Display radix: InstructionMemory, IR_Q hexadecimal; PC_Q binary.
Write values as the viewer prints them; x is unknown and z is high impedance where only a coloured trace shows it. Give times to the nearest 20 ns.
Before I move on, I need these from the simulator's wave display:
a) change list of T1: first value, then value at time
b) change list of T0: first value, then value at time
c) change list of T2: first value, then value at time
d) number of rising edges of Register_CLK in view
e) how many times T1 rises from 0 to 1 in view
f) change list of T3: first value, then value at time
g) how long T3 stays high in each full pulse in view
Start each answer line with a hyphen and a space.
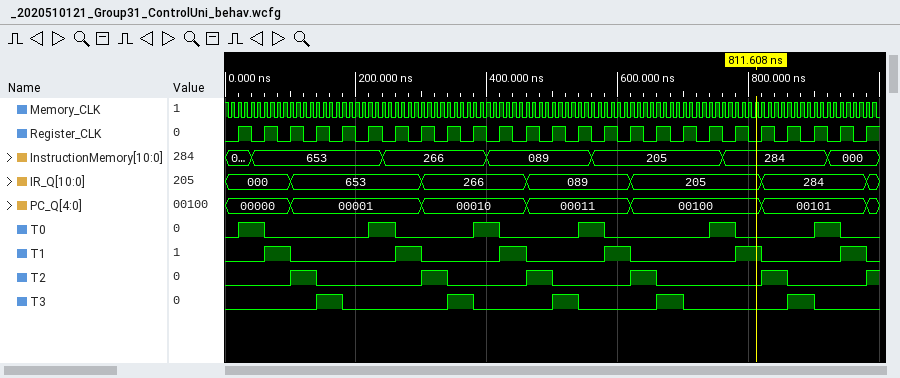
- 0, 1 at 60 ns, 0 at 100 ns, 1 at 260 ns, 0 at 300 ns, 1 at 420 ns, 0 at 460 ns, 1 at 580 ns, 0 at 620 ns, 1 at 780 ns, 0 at 820 ns, 1 at 940 ns, 0 at 980 ns
- 0, 1 at 20 ns, 0 at 60 ns, 1 at 220 ns, 0 at 260 ns, 1 at 380 ns, 0 at 420 ns, 1 at 540 ns, 0 at 580 ns, 1 at 740 ns, 0 at 780 ns, 1 at 900 ns, 0 at 940 ns
- 0, 1 at 100 ns, 0 at 140 ns, 1 at 300 ns, 0 at 340 ns, 1 at 460 ns, 0 at 500 ns, 1 at 620 ns, 0 at 660 ns, 1 at 820 ns, 0 at 860 ns, 1 at 980 ns
- 25
- 6
- 0, 1 at 140 ns, 0 at 180 ns, 1 at 340 ns, 0 at 380 ns, 1 at 500 ns, 0 at 540 ns, 1 at 660 ns, 0 at 700 ns, 1 at 860 ns, 0 at 900 ns
- 40 ns, 40 ns, 40 ns, 40 ns, 40 ns
